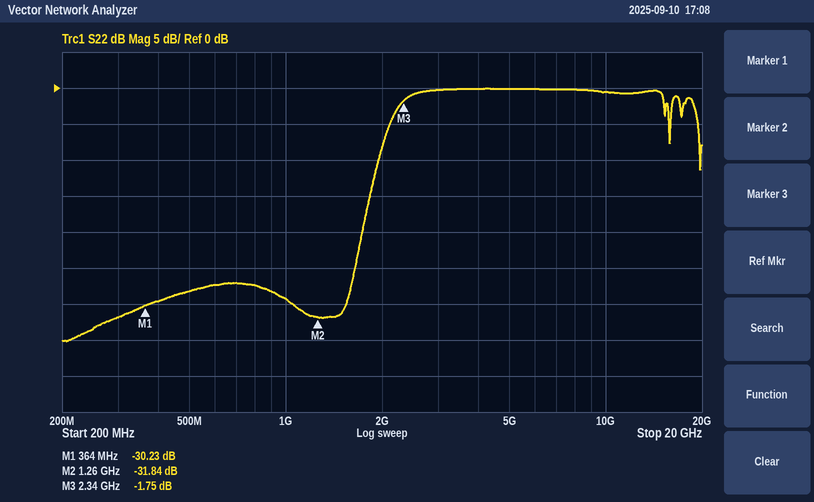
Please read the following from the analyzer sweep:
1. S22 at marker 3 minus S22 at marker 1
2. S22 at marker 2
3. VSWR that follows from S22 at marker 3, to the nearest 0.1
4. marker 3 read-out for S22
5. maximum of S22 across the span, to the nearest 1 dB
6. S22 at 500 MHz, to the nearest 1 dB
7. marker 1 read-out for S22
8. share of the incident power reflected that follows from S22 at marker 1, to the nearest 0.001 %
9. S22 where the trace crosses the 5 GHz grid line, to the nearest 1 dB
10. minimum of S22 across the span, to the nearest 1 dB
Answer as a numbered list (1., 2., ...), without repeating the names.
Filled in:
1. 28.48 dB
2. -31.84 dB
3. 10.0
4. -1.75 dB
5. 0 dB
6. -28 dB
7. -30.23 dB
8. 0.095 %
9. 0 dB
10. -35 dB
